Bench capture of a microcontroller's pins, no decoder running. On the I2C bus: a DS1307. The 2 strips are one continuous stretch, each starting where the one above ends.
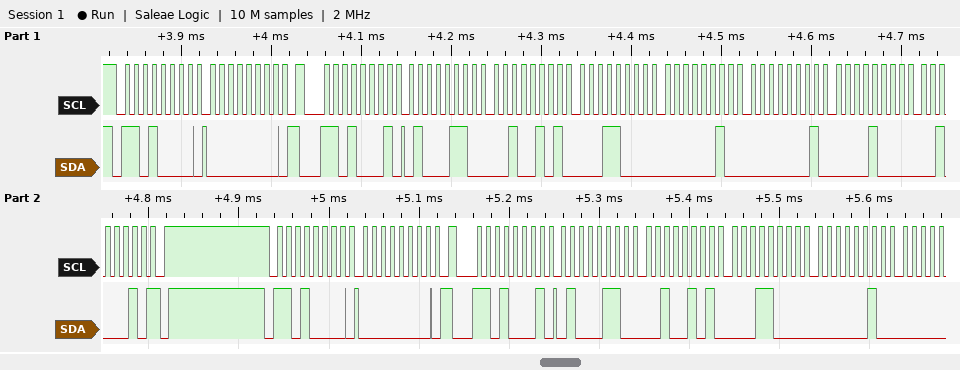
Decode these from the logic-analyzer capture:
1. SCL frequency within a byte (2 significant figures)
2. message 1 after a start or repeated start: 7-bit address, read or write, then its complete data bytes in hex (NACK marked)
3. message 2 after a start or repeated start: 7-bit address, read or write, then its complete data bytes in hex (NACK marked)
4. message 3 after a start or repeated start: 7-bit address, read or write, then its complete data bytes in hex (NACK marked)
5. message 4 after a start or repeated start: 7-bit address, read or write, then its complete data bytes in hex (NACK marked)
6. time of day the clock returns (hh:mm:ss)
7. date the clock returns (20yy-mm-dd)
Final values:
100 kHz
0x68 write: 00
0x68 read: 46 25 18 02 01 08 22 NACK
0x68 write: 00
0x68 read: 46 25 18 02
18:25:46
2022-08-01
